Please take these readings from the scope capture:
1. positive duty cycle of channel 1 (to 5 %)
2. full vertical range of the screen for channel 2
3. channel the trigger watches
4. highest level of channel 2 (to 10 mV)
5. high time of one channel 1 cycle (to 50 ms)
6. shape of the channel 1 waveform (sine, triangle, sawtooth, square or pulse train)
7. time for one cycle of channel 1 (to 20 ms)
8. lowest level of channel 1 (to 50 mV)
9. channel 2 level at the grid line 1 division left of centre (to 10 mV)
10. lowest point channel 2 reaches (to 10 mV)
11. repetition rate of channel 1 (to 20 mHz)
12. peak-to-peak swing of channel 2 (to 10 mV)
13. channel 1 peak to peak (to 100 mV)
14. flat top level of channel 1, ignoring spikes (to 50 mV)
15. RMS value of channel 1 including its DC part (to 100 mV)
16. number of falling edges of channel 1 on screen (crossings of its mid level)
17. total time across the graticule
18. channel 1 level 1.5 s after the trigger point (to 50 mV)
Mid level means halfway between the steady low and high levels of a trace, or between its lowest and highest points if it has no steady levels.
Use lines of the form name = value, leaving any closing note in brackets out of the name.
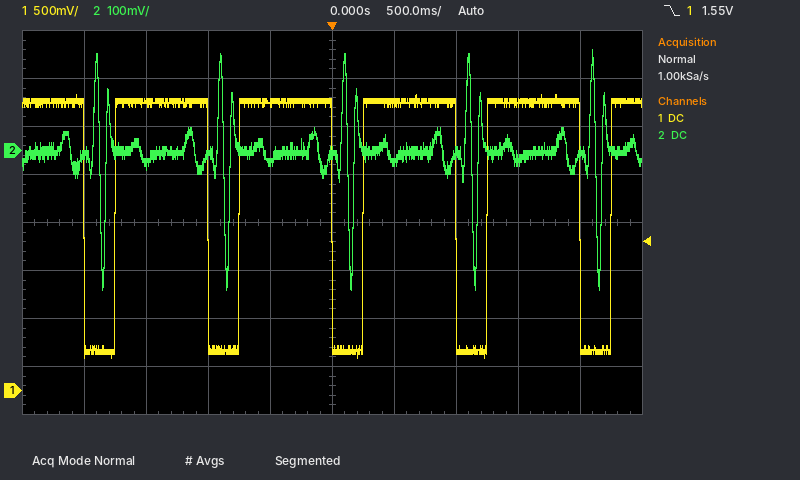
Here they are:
positive duty cycle of channel 1 = 75 %
full vertical range of the screen for channel 2 = 800 mV
channel the trigger watches = channel 1
highest level of channel 2 = 210 mV
high time of one channel 1 cycle = 750 ms
shape of the channel 1 waveform = pulse train
time for one cycle of channel 1 = 1.00 s
lowest level of channel 1 = 350 mV
channel 2 level at the grid line 1 division left of centre = -20 mV
lowest point channel 2 reaches = -290 mV
repetition rate of channel 1 = 1.00 Hz
peak-to-peak swing of channel 2 = 500 mV
channel 1 peak to peak = 2.70 V
flat top level of channel 1, ignoring spikes = 3.00 V
RMS value of channel 1 including its DC part = 2.6 V
number of falling edges of channel 1 on screen = 5
total time across the graticule = 5 s
channel 1 level 1.5 s after the trigger point = 3.00 V
